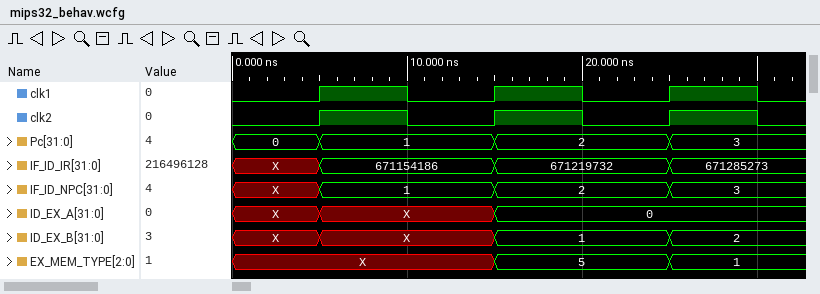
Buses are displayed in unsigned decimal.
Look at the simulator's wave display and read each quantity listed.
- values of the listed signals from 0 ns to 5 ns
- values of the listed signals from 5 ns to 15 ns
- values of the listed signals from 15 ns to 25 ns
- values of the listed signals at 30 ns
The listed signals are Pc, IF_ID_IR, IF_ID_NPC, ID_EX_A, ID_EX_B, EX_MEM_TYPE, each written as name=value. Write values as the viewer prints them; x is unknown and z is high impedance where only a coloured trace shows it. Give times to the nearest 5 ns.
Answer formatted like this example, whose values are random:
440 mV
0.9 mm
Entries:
Pc=0, IF_ID_IR=X, IF_ID_NPC=X, ID_EX_A=X, ID_EX_B=X, EX_MEM_TYPE=X
Pc=1, IF_ID_IR=671154186, IF_ID_NPC=1, ID_EX_A=X, ID_EX_B=X, EX_MEM_TYPE=X
Pc=2, IF_ID_IR=671219732, IF_ID_NPC=2, ID_EX_A=0, ID_EX_B=1, EX_MEM_TYPE=5
Pc=3, IF_ID_IR=671285273, IF_ID_NPC=3, ID_EX_A=0, ID_EX_B=2, EX_MEM_TYPE=1
